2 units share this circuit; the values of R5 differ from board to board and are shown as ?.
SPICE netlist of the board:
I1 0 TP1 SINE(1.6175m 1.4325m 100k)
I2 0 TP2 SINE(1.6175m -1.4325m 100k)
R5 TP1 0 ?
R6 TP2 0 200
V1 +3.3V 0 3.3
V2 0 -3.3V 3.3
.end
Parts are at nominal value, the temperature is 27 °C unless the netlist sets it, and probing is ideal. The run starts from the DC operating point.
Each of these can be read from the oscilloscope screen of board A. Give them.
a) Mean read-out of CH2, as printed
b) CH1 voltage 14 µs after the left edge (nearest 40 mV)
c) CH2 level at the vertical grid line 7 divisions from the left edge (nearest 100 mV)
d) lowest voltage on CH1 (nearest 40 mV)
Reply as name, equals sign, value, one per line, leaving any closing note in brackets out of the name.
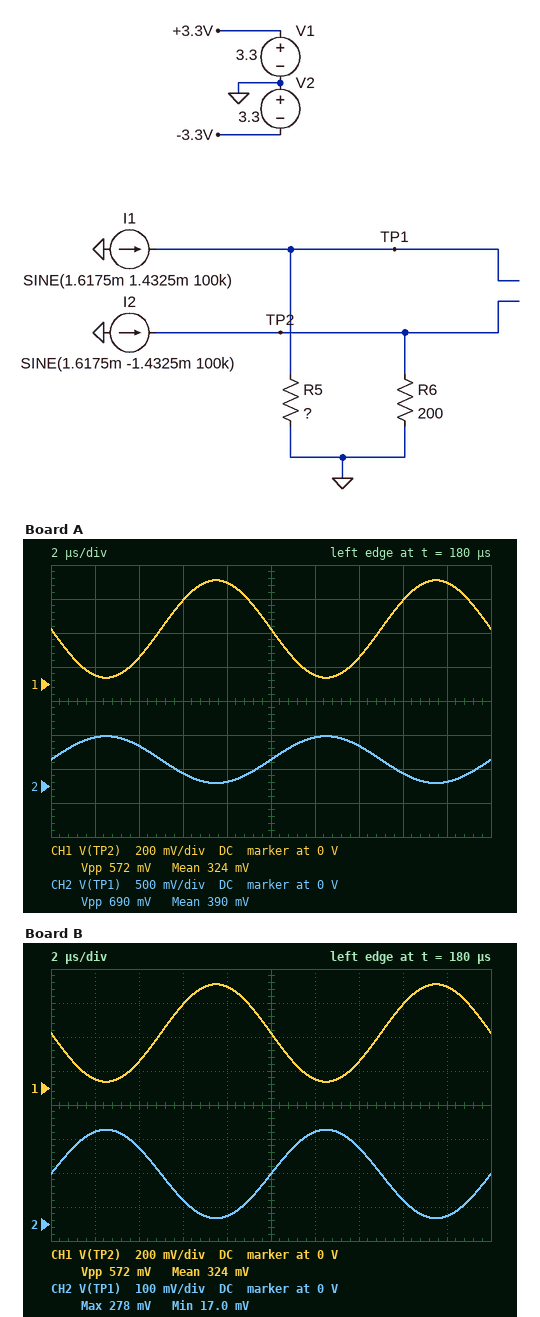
Mean read-out of CH2, as printed = 390 mV
CH1 voltage 14 µs after the left edge = 160 mV
CH2 level at the vertical grid line 7 divisions from the left edge = 600 mV
lowest voltage on CH1 = 40 mV
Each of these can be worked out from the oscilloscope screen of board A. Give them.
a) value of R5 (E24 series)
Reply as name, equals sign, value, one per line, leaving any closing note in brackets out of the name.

value of R5 = 240 Ω
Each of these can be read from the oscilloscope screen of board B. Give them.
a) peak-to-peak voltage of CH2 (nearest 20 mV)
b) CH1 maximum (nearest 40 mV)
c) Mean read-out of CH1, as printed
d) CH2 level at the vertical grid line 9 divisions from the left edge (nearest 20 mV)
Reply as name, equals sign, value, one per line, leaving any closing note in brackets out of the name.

peak-to-peak voltage of CH2 = 260 mV
CH1 maximum = 600 mV
Mean read-out of CH1, as printed = 324 mV
CH2 level at the vertical grid line 9 divisions from the left edge = 20 mV
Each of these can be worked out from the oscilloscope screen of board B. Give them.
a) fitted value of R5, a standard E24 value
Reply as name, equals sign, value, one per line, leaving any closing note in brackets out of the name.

fitted value of R5, a standard E24 value = 91 Ω
